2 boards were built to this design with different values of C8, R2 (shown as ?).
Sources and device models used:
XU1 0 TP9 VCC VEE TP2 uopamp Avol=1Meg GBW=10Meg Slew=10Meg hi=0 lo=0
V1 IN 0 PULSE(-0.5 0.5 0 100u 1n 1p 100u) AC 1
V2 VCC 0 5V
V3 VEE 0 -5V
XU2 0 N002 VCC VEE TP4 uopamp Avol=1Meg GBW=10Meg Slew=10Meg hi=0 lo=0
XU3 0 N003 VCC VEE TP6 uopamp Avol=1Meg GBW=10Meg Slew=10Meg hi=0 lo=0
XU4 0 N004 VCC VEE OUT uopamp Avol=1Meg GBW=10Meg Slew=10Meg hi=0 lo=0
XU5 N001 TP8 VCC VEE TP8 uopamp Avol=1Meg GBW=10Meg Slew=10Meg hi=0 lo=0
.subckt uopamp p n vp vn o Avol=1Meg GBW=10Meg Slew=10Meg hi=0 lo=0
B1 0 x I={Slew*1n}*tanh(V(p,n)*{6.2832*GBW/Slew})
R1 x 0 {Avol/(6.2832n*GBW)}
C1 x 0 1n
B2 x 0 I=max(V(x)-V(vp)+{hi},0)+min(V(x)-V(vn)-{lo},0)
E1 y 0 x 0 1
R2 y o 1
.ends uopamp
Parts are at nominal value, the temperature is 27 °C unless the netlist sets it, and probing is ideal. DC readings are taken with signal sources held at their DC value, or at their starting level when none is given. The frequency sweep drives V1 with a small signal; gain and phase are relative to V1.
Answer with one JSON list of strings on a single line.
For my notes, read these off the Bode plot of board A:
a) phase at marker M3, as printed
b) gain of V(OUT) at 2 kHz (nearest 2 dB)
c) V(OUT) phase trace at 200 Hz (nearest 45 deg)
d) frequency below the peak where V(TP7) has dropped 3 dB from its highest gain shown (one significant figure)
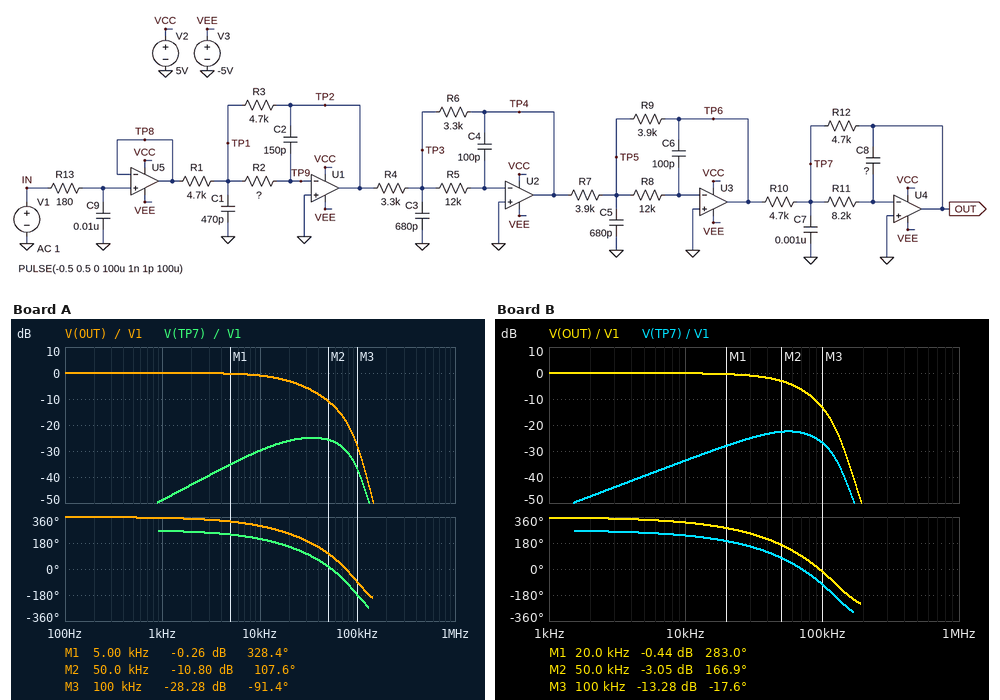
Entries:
["-91.4 deg", "0 dB", "360 deg", "10 kHz"]
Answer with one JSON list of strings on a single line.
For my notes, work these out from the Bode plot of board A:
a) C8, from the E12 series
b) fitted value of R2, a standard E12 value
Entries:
["68 pF", "27 kΩ"]
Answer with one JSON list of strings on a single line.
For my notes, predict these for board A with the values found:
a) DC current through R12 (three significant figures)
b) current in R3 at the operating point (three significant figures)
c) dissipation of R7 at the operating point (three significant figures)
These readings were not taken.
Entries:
["106 µA", "106 µA", "64.1 µW"]
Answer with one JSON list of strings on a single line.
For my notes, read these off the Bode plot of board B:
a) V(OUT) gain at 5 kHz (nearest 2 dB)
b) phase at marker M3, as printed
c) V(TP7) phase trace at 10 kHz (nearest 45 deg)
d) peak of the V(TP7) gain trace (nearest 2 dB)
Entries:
["0 dB", "-17.6 deg", "225 deg", "-22 dB"]
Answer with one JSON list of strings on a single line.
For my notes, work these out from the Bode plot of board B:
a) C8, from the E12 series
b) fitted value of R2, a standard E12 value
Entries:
["39 pF", "5.6 kΩ"]
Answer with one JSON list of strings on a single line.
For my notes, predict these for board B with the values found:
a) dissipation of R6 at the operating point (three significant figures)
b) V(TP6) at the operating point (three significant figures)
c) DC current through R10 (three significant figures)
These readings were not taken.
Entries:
["75.8 µW", "500 mV", "106 µA"]
